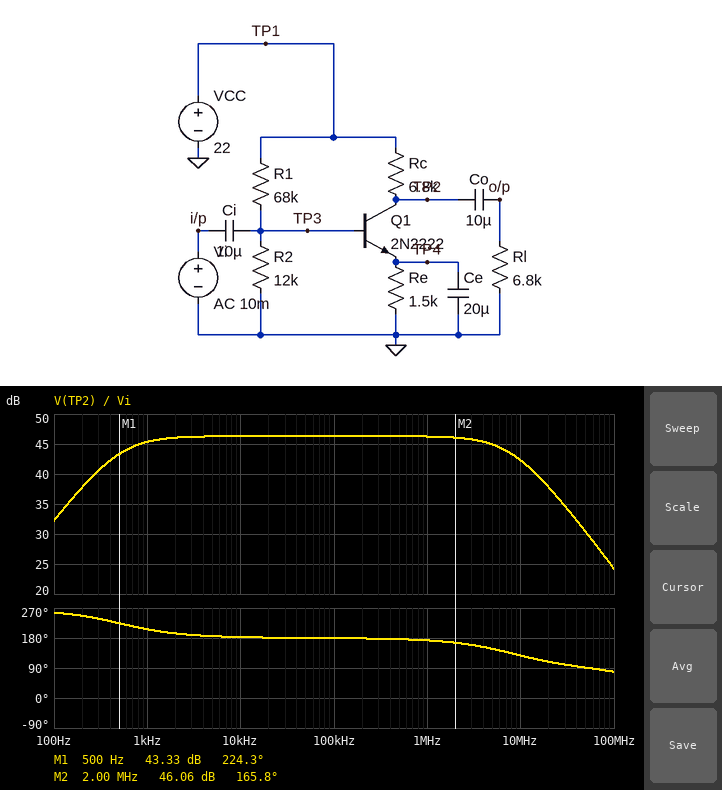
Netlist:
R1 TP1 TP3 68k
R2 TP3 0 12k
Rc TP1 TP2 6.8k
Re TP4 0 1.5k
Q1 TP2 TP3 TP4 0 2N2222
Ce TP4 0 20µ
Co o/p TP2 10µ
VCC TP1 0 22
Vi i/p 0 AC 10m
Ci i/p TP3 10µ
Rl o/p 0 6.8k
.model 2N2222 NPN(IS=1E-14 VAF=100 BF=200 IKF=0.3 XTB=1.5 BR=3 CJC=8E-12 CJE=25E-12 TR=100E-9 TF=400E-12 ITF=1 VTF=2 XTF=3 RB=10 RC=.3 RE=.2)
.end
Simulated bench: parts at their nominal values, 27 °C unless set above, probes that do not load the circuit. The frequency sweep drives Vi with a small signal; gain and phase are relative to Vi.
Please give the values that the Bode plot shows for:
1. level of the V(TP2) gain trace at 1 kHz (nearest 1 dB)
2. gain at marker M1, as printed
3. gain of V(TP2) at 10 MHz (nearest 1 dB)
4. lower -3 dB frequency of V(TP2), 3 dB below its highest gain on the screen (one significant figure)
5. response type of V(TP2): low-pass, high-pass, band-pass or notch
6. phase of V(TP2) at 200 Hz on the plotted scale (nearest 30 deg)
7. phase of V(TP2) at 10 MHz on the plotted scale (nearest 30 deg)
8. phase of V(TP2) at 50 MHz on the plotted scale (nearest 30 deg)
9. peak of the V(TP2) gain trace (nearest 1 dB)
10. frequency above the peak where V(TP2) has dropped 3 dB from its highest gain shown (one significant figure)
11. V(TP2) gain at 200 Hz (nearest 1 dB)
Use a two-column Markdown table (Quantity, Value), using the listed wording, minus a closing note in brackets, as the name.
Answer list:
| Quantity | Value |
|---|---|
| level of the V(TP2) gain trace at 1 kHz | 45 dB |
| gain at marker M1, as printed | 43.33 dB |
| gain of V(TP2) at 10 MHz | 42 dB |
| lower -3 dB frequency of V(TP2), 3 dB below its highest gain on the screen | 500 Hz |
| response type of V(TP2): low-pass, high-pass, band-pass or notch | band-pass |
| phase of V(TP2) at 200 Hz on the plotted scale | 240 deg |
| phase of V(TP2) at 10 MHz on the plotted scale | 120 deg |
| phase of V(TP2) at 50 MHz on the plotted scale | 90 deg |
| peak of the V(TP2) gain trace | 46 dB |
| frequency above the peak where V(TP2) has dropped 3 dB from its highest gain shown | 8 MHz |
| V(TP2) gain at 200 Hz | 38 dB |
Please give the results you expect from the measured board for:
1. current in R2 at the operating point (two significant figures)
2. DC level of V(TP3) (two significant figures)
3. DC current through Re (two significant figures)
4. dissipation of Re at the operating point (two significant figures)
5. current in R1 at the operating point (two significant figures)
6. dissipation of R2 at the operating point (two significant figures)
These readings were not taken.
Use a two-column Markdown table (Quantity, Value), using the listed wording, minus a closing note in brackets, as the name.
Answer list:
| Quantity | Value |
|---|---|
| current in R2 at the operating point | 270 µA |
| DC level of V(TP3) | 3.2 V |
| DC current through Re | 1.7 mA |
| dissipation of Re at the operating point | 4.3 mW |
| current in R1 at the operating point | 280 µA |
| dissipation of R2 at the operating point | 860 µW |
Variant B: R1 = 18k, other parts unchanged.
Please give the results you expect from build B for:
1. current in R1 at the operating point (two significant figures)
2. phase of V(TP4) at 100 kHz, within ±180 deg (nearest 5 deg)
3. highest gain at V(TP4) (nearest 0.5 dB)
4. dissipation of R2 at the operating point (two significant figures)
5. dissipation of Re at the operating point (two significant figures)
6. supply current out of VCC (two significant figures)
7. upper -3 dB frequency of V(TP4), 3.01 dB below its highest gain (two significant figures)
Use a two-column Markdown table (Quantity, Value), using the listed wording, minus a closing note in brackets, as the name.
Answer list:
| Quantity | Value |
|---|---|
| current in R1 at the operating point | 930 µA |
| phase of V(TP4) at 100 kHz, within ±180 deg | -85 deg |
| highest gain at V(TP4) | -9.5 dB |
| dissipation of R2 at the operating point | 2.3 mW |
| dissipation of Re at the operating point | 14 mW |
| supply current out of VCC | 3.5 mA |
| upper -3 dB frequency of V(TP4), 3.01 dB below its highest gain | 740 Hz |
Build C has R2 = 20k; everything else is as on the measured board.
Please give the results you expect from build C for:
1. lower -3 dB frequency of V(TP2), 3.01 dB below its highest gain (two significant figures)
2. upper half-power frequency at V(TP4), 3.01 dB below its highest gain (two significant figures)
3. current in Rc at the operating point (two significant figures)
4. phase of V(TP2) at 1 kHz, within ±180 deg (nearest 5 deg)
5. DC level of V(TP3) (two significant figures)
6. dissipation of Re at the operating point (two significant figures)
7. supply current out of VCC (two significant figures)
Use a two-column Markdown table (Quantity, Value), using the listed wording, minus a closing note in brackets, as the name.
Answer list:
| Quantity | Value |
|---|---|
| lower -3 dB frequency of V(TP2), 3.01 dB below its highest gain | 540 Hz |
| upper half-power frequency at V(TP4), 3.01 dB below its highest gain | 550 Hz |
| current in Rc at the operating point | 2.6 mA |
| phase of V(TP2) at 1 kHz, within ±180 deg | -150 deg |
| DC level of V(TP3) | 4.7 V |
| dissipation of Re at the operating point | 11 mW |
| supply current out of VCC | 2.9 mA |
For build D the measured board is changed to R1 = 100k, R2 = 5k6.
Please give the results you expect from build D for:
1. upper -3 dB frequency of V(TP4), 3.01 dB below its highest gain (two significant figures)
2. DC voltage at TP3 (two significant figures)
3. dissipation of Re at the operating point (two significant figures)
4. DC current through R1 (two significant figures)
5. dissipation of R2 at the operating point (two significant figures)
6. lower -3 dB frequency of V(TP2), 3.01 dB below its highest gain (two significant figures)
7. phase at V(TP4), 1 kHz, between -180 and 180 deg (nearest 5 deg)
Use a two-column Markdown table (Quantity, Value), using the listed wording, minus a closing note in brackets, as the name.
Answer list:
| Quantity | Value |
|---|---|
| upper -3 dB frequency of V(TP4), 3.01 dB below its highest gain | 120 Hz |
| DC voltage at TP3 | 1.2 V |
| dissipation of Re at the operating point | 190 µW |
| DC current through R1 | 210 µA |
| dissipation of R2 at the operating point | 240 µW |
| lower -3 dB frequency of V(TP2), 3.01 dB below its highest gain | 110 Hz |
| phase at V(TP4), 1 kHz, between -180 and 180 deg | -85 deg |
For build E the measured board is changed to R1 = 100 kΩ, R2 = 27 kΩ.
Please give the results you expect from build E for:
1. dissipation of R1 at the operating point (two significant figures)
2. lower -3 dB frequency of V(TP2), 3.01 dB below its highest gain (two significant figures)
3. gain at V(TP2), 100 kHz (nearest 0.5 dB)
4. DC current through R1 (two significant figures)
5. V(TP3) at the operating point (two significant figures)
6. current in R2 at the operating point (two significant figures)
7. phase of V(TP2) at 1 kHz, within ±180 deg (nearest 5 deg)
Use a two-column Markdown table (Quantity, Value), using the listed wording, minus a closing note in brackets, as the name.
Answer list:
| Quantity | Value |
|---|---|
| dissipation of R1 at the operating point | 3.1 mW |
| lower -3 dB frequency of V(TP2), 3.01 dB below its highest gain | 700 Hz |
| gain at V(TP2), 100 kHz | 49.5 dB |
| DC current through R1 | 180 µA |
| V(TP3) at the operating point | 4.4 V |
| current in R2 at the operating point | 160 µA |
| phase of V(TP2) at 1 kHz, within ±180 deg | -145 deg |
